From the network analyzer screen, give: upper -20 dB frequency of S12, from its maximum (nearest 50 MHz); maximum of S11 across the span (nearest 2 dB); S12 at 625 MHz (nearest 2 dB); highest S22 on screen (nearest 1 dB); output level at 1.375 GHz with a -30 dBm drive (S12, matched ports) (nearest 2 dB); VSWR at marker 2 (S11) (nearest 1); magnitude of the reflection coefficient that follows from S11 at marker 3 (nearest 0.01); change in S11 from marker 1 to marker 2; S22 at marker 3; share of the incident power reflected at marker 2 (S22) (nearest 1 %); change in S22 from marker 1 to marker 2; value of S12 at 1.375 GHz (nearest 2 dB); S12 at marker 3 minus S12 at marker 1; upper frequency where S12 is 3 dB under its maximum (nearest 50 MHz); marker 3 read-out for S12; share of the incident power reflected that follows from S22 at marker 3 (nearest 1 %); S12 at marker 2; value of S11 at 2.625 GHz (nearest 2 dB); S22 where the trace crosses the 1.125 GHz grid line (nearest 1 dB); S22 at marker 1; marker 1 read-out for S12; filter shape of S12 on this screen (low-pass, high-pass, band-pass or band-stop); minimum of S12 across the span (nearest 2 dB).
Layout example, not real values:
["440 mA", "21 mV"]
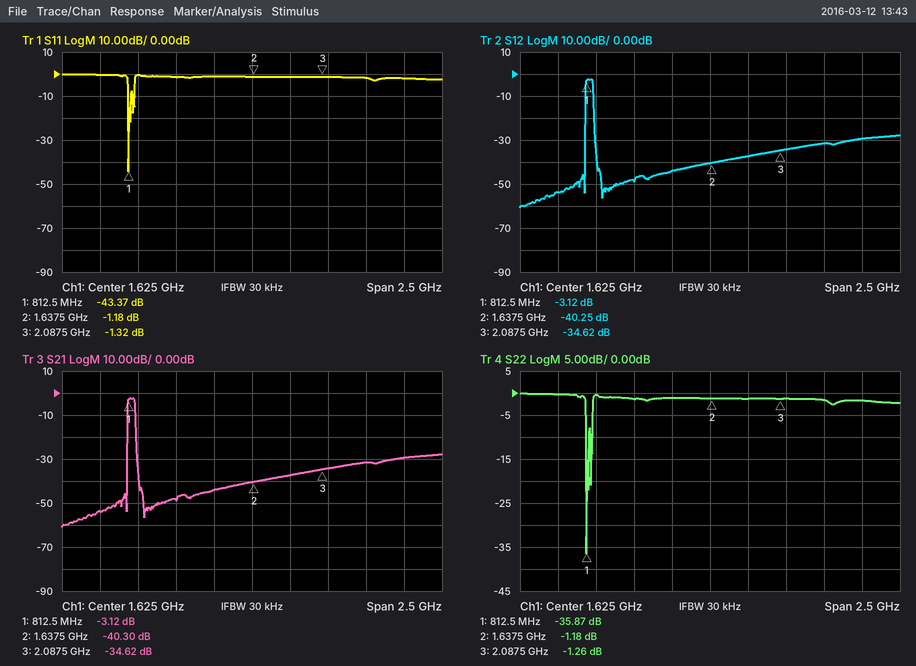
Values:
["850 MHz", "0 dB", "-54 dB", "0 dB", "-74 dBm", "15", "0.86", "42.19 dB", "-1.26 dB", "76 %", "34.69 dB", "-44 dB", "-31.50 dB", "850 MHz", "-34.62 dB", "75 %", "-40.25 dB", "-2 dB", "-1 dB", "-35.87 dB", "-3.12 dB", "band-pass", "-60 dB"]
